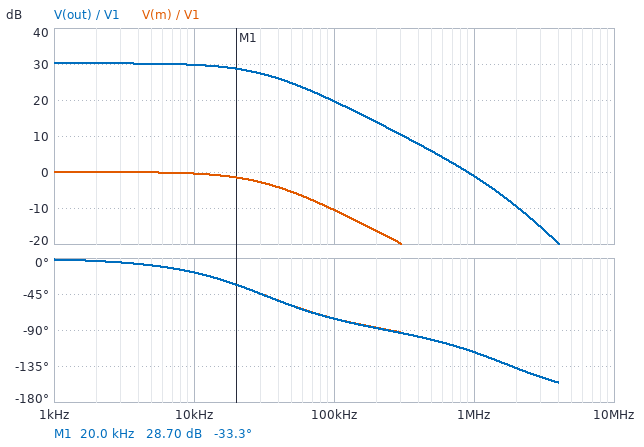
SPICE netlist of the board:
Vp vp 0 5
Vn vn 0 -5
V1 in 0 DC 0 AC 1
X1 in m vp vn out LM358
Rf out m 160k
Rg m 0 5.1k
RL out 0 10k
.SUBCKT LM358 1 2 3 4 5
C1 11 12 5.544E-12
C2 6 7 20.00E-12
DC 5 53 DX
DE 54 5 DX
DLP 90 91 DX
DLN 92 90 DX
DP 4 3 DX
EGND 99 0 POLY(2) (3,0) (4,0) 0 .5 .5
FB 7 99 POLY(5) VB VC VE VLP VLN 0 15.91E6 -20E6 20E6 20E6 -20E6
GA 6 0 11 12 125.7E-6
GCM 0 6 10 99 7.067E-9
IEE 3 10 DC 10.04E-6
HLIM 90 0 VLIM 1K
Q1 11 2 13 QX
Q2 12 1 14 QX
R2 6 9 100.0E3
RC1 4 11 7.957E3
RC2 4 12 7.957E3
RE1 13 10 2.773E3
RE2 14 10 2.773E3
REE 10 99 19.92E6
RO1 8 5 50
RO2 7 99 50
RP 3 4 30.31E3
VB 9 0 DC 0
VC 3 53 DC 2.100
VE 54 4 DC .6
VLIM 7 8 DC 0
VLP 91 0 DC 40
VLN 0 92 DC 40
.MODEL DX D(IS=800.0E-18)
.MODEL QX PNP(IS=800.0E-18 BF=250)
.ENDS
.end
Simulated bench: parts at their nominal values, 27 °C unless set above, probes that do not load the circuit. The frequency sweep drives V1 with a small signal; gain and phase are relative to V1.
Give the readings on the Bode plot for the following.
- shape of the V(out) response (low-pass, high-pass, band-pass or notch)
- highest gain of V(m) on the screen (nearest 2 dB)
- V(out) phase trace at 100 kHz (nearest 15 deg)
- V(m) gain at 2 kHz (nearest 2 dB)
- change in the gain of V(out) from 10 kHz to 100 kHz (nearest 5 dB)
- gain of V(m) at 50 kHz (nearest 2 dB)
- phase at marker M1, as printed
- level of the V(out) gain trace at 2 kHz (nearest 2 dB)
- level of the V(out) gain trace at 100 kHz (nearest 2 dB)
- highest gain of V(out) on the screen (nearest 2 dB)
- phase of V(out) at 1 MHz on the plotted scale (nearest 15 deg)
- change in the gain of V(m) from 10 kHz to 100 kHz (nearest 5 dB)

low-pass
0 dB
-75 deg
0 dB
-10 dB
-6 dB
-33.3 deg
30 dB
20 dB
30 dB
-120 deg
-10 dB
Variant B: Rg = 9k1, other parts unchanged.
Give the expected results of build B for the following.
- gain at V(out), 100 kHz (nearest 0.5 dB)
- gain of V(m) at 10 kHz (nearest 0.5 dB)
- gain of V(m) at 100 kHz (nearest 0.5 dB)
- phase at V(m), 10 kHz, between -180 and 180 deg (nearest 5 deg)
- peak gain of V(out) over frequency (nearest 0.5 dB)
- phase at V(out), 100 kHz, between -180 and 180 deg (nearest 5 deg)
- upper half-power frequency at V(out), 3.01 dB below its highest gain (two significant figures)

19.0 dB
0 dB
-6.5 dB
-10 deg
25.5 dB
-65 deg
55 kHz
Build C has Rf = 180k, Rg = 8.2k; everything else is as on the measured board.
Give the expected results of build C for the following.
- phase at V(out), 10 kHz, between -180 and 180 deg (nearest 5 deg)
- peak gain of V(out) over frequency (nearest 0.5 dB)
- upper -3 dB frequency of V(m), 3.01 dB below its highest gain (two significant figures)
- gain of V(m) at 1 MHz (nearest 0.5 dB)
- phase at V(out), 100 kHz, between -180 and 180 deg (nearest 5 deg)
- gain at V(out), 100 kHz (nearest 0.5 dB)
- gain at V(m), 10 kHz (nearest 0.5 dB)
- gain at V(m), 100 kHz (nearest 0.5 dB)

-15 deg
27.0 dB
44 kHz
-28.5 dB
-70 deg
19.5 dB
0 dB
-8.0 dB
